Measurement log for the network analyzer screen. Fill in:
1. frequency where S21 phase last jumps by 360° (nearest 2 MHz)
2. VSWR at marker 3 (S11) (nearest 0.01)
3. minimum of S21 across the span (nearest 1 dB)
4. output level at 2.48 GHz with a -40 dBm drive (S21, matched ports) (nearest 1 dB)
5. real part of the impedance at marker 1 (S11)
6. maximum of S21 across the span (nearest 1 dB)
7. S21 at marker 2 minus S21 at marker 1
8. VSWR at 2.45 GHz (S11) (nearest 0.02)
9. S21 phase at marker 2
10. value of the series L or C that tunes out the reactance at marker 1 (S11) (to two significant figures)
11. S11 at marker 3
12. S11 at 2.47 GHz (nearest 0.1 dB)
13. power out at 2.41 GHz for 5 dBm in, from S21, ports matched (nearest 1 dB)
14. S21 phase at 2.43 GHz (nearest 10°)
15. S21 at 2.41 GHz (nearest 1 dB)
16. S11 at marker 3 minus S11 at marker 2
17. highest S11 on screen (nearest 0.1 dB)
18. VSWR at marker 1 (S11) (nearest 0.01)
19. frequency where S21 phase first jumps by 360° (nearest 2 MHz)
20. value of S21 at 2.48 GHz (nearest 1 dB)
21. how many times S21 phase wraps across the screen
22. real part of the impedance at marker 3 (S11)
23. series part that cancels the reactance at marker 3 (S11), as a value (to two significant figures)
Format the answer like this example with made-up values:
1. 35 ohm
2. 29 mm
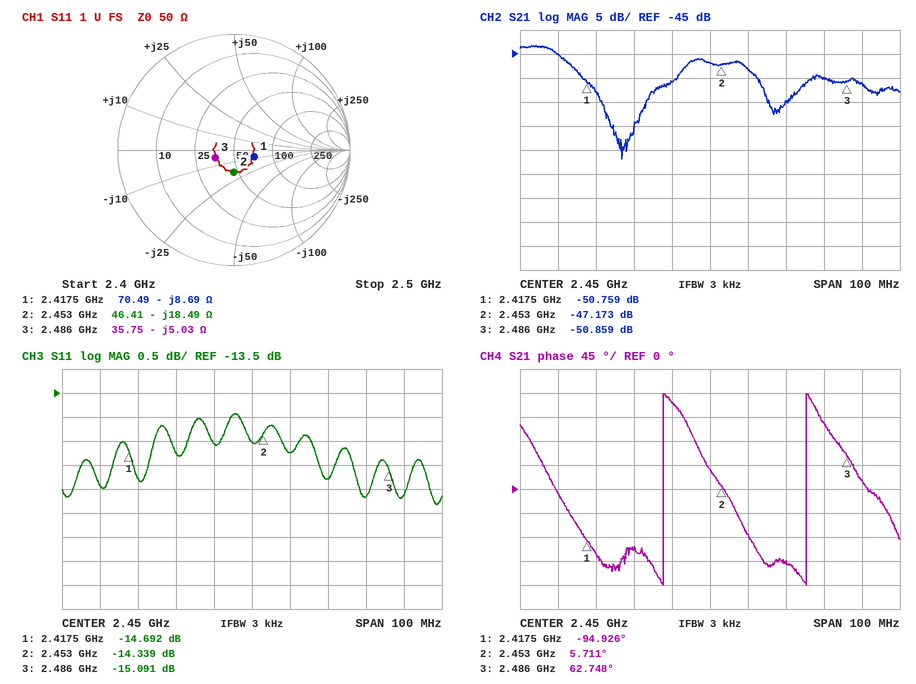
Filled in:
1. 2.476 GHz
2. 1.43
3. -67 dB
4. -90 dBm
5. 70.49 Ω
6. -43 dB
7. 3.586 dB
8. 1.46
9. 5.711°
10. 570 pH
11. -15.091 dB
12. -15.3 dB
13. -40 dBm
14. -110°
15. -45 dB
16. -0.752 dB
17. -13.9 dB
18. 1.45
19. 2.438 GHz
20. -50 dB
21. 2
22. 35.75 Ω
23. 320 pH
